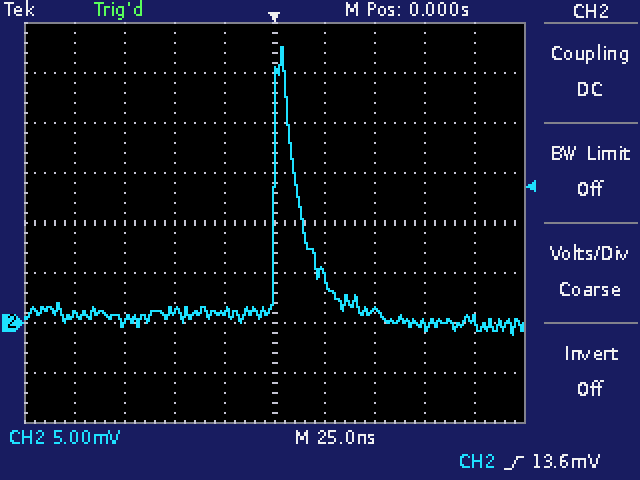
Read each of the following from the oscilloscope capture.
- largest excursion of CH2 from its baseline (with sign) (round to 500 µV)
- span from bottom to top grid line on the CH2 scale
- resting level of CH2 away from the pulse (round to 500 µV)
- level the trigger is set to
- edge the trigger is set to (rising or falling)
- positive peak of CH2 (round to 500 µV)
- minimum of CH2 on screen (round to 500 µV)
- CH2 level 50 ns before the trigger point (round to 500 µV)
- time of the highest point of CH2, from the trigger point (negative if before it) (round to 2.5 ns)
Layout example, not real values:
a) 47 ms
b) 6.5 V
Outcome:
a) +26.5 mV
b) 40 mV
c) 1.0 mV
d) 13.6 mV
e) rising
f) 27.5 mV
g) -1.0 mV
h) 1.0 mV
i) +5.0 ns
